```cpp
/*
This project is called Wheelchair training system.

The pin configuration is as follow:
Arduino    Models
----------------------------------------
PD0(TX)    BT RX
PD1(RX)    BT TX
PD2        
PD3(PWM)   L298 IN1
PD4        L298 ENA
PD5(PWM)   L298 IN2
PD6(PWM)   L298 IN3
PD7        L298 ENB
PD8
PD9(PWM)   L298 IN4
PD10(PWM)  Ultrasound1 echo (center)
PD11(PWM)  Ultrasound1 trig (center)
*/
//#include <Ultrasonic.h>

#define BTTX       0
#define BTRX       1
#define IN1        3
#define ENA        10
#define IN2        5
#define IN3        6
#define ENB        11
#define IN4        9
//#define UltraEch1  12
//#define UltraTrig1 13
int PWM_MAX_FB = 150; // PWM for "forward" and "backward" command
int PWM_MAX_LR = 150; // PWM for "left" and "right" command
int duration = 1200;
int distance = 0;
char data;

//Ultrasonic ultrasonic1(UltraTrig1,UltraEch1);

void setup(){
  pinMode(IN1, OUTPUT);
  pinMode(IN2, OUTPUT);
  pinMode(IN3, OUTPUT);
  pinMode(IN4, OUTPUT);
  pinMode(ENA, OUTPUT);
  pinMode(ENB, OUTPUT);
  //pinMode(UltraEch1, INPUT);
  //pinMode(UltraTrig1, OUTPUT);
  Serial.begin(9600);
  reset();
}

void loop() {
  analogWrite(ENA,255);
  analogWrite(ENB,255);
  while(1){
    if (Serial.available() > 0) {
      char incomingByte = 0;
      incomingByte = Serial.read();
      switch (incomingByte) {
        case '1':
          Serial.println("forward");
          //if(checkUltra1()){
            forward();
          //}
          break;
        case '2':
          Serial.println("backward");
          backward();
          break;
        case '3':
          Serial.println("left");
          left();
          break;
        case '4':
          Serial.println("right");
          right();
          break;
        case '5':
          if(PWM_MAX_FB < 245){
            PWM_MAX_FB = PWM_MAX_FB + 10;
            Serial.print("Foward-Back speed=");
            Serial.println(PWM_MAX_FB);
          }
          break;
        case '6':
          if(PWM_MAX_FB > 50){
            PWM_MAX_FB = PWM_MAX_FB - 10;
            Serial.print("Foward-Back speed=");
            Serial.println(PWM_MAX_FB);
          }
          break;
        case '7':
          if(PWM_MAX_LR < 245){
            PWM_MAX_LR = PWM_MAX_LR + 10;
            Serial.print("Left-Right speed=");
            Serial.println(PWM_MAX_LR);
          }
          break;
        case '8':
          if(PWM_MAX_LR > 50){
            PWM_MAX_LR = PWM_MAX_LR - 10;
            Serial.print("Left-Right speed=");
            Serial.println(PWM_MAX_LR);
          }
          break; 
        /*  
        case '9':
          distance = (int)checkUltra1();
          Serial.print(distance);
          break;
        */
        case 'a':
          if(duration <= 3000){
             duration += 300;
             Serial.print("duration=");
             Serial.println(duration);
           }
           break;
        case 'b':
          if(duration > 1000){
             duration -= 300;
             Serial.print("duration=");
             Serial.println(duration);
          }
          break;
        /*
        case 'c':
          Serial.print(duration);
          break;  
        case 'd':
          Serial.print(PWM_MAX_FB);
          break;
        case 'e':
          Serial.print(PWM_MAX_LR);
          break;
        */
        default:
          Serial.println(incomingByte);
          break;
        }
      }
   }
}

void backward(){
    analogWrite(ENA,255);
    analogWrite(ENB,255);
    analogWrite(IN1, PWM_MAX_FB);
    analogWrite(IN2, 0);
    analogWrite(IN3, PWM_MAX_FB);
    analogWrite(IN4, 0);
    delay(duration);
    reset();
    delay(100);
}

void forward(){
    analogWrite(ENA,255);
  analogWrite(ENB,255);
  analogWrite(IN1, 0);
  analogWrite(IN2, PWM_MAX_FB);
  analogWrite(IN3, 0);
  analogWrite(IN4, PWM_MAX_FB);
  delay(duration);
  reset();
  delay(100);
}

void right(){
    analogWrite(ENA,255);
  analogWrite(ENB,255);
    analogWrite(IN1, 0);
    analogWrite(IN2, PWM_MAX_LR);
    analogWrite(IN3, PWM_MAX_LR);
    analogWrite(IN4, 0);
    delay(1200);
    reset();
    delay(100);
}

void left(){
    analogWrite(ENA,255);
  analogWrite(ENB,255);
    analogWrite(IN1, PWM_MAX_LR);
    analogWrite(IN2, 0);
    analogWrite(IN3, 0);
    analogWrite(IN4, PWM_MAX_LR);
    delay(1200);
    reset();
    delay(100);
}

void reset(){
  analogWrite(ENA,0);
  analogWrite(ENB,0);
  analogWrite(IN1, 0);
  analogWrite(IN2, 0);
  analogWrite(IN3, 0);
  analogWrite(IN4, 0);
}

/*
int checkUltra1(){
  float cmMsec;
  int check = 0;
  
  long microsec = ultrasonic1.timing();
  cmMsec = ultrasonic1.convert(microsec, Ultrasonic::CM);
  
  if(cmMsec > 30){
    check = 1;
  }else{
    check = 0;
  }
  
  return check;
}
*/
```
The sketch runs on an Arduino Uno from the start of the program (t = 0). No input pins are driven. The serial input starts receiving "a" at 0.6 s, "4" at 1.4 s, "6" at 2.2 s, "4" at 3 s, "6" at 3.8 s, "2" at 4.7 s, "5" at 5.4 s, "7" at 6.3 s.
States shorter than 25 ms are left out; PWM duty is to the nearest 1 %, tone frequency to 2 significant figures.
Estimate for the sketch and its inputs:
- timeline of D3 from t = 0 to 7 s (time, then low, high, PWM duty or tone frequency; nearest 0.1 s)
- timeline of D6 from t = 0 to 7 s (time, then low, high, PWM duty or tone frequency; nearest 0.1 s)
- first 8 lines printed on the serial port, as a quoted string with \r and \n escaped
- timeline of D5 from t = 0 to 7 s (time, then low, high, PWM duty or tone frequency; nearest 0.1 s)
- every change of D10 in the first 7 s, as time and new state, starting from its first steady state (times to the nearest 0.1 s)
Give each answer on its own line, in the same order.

0 s low; 4.7 s PWM 51 %; 6.2 s low
0 s low; 1.4 s PWM 59 %; 2.6 s low; 3 s PWM 59 %; 4.2 s low; 4.7 s PWM 51 %; 6.2 s low
"duration=1500\r\nright\r\nFoward-Back speed=140\r\nright\r\nFoward-Back speed=130\r\nbackward\r\nFoward-Back speed=140\r\nLeft-Right speed=160\r\n"
0 s low; 1.4 s PWM 59 %; 2.6 s low; 3 s PWM 59 %; 4.2 s low
0 s high; 2.6 s low; 3 s high; 4.2 s low; 4.7 s high; 6.2 s low
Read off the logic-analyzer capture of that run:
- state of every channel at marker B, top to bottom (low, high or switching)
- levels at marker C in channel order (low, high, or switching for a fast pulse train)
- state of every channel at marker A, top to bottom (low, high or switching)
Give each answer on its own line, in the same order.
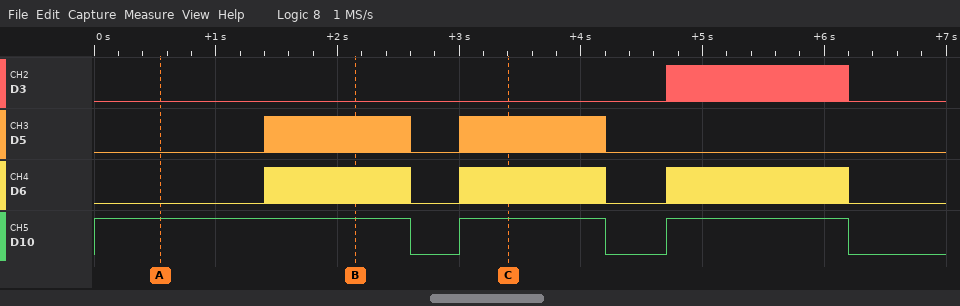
D3 low, D5 switching, D6 switching, D10 high
D3 low, D5 switching, D6 switching, D10 high
D3 low, D5 low, D6 low, D10 high
